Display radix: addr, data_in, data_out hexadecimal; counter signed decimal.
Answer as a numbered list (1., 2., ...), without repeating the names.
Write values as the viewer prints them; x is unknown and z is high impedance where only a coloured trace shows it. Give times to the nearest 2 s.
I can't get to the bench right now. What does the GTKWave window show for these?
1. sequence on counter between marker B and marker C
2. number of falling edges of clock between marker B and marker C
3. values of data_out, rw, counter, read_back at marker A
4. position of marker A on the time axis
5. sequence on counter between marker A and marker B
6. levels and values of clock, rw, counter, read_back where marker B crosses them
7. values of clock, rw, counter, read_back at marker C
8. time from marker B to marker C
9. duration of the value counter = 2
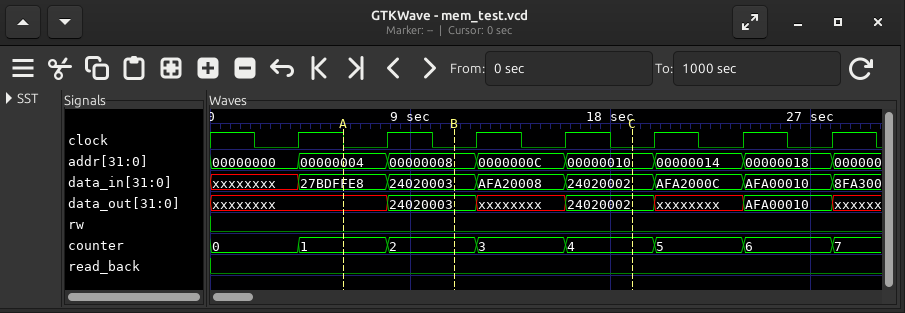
1. 2, 3, 4
2. 2
3. data_out=xxxxxxxx, rw=0, counter=1, read_back=0
4. 6 s
5. 1, 2
6. clock=0, rw=0, counter=2, read_back=0
7. clock=0, rw=0, counter=4, read_back=0
8. 8 s
9. 4 s
